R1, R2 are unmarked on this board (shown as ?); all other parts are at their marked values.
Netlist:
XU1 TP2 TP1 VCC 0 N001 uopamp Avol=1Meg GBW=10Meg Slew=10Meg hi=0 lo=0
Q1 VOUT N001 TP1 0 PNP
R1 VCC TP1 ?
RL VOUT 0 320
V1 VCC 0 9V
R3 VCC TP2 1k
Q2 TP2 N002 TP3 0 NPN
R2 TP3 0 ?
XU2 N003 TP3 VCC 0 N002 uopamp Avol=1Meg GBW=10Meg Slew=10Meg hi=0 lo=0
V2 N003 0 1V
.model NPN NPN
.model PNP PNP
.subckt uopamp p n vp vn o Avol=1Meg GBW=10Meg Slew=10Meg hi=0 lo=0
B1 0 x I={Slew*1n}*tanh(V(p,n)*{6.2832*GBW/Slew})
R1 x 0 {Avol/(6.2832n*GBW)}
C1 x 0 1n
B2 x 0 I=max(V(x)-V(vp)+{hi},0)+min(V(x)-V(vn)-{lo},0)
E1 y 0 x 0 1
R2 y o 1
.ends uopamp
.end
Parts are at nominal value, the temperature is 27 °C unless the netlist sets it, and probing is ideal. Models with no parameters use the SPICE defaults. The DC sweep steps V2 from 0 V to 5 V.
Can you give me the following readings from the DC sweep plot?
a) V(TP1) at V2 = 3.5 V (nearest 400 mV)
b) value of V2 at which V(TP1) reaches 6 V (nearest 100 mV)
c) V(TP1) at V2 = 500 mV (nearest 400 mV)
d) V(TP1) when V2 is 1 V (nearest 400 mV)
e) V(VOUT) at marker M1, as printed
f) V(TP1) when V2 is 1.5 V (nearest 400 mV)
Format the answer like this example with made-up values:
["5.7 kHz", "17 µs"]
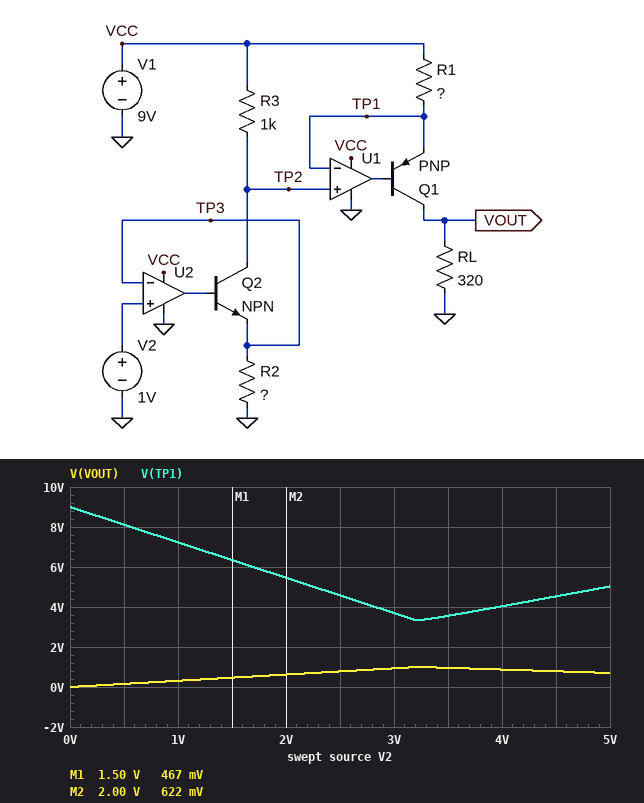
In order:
["3.6 V", "1.7 V", "8.0 V", "7.2 V", "467 mV", "6.4 V"]
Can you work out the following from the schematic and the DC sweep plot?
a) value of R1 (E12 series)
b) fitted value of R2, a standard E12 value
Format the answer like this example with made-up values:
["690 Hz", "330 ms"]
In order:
["1.8 kΩ", "560 Ω"]
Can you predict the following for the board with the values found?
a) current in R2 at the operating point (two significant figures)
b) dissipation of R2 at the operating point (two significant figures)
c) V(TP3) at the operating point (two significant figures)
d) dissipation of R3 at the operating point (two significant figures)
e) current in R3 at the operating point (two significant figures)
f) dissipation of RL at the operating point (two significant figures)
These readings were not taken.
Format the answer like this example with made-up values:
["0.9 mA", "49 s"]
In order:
["1.8 mA", "1.8 mW", "1.0 V", "3.1 mW", "1.8 mA", "300 µW"]
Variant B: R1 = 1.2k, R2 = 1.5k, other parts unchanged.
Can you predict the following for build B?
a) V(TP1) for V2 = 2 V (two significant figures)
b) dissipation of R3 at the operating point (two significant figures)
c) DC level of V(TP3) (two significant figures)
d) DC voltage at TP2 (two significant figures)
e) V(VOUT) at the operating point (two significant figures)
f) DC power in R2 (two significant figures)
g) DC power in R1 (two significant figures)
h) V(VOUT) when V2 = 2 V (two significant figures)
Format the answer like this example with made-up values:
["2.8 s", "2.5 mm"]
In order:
["7.7 V", "440 µW", "1.0 V", "8.3 V", "170 mV", "670 µW", "360 µW", "350 mV"]
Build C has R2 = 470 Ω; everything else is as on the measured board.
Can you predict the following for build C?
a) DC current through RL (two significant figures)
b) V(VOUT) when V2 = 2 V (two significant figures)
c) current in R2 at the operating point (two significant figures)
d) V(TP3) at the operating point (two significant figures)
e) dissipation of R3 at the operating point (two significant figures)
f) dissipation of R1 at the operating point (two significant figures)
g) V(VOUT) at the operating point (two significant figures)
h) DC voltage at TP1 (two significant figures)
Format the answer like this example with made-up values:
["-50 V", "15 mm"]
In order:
["1.2 mA", "740 mV", "2.1 mA", "1.0 V", "4.4 mW", "2.5 mW", "370 mV", "6.9 V"]
